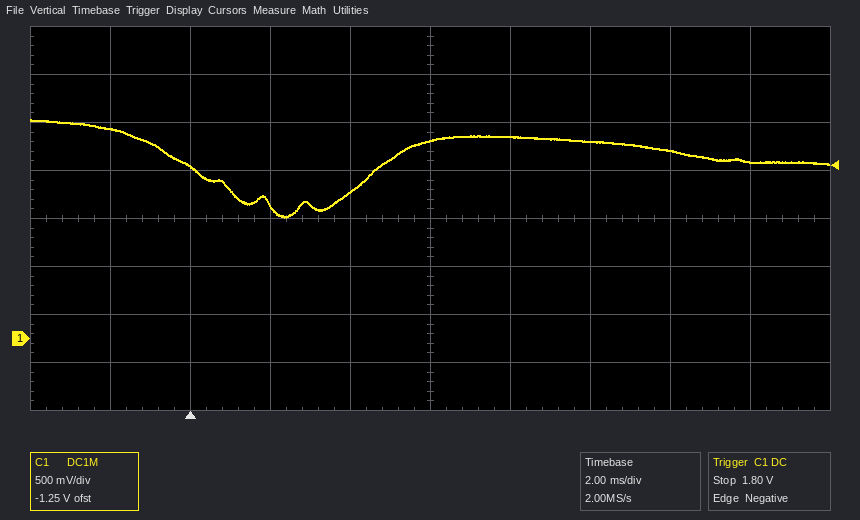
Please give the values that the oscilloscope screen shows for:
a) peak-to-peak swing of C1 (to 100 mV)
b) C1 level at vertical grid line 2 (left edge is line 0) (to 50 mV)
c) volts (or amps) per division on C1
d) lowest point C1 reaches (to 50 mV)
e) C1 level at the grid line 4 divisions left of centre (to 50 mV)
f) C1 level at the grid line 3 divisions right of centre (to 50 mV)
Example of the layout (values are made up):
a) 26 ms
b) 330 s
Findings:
a) 1.00 V
b) 1.80 V
c) 500 mV
d) 1.25 V
e) 2.20 V
f) 1.95 V
